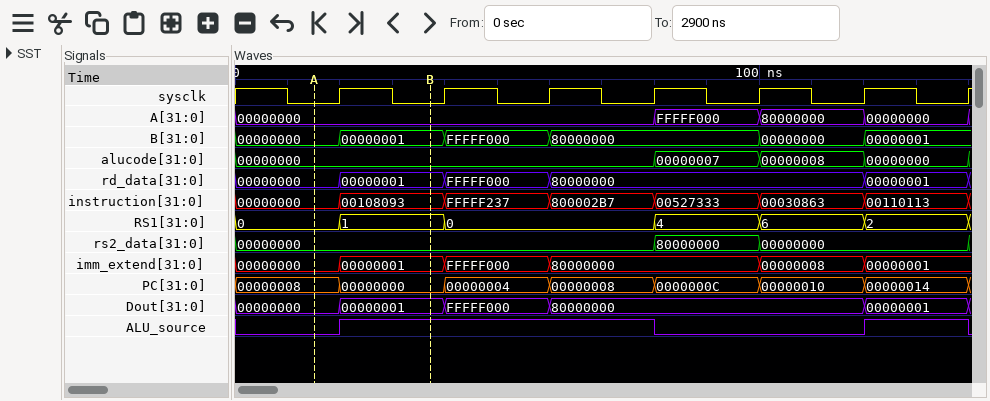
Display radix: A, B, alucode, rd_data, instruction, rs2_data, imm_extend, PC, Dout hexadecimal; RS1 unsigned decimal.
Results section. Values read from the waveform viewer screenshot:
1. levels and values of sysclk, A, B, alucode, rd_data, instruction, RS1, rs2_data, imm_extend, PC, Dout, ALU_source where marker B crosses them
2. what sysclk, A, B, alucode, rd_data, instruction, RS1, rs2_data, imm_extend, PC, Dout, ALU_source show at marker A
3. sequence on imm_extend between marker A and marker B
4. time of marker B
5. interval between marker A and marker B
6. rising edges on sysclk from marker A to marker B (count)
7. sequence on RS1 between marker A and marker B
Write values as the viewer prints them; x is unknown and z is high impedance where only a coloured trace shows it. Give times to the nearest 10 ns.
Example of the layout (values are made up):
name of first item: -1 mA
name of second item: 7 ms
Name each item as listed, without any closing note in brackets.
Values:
levels and values of sysclk, A, B, alucode, rd_data, instruction, RS1, rs2_data, imm_extend, PC, Dout, ALU_source where marker B crosses them: sysclk=0, A=00000000, B=00000001, alucode=00000000, rd_data=00000001, instruction=00108093, RS1=1, rs2_data=00000000, imm_extend=00000001, PC=00000000, Dout=00000001, ALU_source=1
what sysclk, A, B, alucode, rd_data, instruction, RS1, rs2_data, imm_extend, PC, Dout, ALU_source show at marker A: sysclk=0, A=00000000, B=00000000, alucode=00000000, rd_data=00000000, instruction=00000000, RS1=0, rs2_data=00000000, imm_extend=00000000, PC=00000008, Dout=00000000, ALU_source=0
sequence on imm_extend between marker A and marker B: 00000000, 00000001
time of marker B: 40 ns
interval between marker A and marker B: 20 ns
rising edges on sysclk from marker A to marker B: 1
sequence on RS1 between marker A and marker B: 0, 1
